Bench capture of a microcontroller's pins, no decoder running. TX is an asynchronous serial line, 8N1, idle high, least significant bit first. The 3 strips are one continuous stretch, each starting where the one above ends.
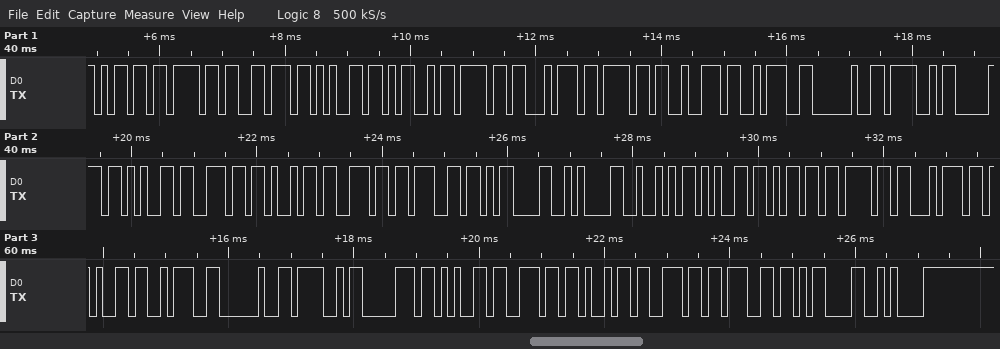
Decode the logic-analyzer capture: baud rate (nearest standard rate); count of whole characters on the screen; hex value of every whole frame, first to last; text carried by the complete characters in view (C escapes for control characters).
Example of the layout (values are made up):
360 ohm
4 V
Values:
9600 baud
37
6D 6F 76 65 4D 6F 74 6F 72 3A 20 4F 70 65 6E 69 6E 67 0D 0A 52 65 6D 6F 74 65 3A 20 4F 70 65 6E 69 6E 67 0D 0A
"moveMotor: Opening\r\nRemote: Opening\r\n"
